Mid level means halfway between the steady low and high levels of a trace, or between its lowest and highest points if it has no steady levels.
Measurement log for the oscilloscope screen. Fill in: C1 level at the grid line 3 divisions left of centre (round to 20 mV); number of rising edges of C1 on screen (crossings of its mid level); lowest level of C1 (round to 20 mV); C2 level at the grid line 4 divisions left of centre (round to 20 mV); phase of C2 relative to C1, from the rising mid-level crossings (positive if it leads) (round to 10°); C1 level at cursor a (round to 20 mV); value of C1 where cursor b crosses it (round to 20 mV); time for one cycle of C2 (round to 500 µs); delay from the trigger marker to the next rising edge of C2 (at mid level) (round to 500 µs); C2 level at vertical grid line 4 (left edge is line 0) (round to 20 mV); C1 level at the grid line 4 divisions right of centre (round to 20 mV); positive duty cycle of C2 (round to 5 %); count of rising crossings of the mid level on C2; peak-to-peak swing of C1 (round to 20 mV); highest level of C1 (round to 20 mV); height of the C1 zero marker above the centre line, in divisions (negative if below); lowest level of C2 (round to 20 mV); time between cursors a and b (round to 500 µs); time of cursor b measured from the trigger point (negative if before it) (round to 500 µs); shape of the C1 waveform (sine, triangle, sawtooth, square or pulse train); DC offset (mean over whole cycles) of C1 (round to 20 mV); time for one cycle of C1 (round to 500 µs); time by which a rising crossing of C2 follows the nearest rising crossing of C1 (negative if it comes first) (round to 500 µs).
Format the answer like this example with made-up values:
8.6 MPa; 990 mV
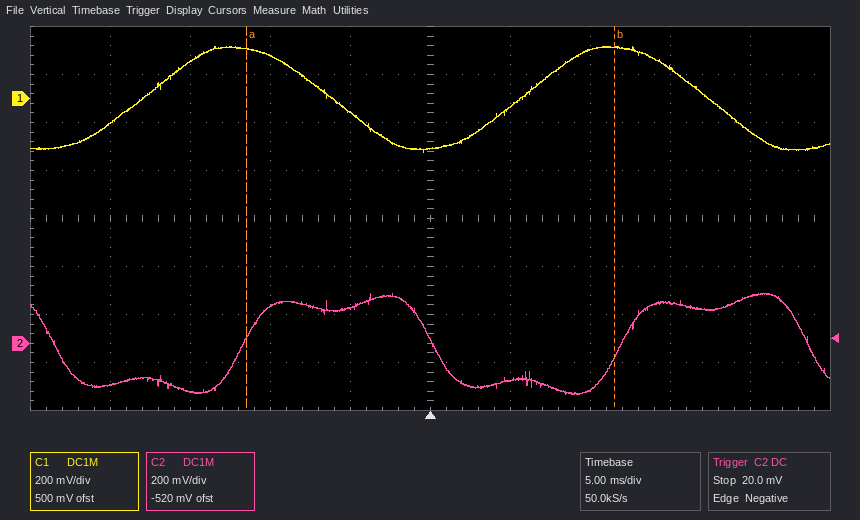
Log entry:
160 mV; 2; -220 mV; -180 mV; -100°; 200 mV; 220 mV; 23.5 ms; 12.0 ms; 140 mV; -140 mV; 50 %; 2; 440 mV; 220 mV; +2.5 div; -220 mV; 23.0 ms; +11.5 ms; sine; 0 mV; 23.5 ms; +6.5 ms
